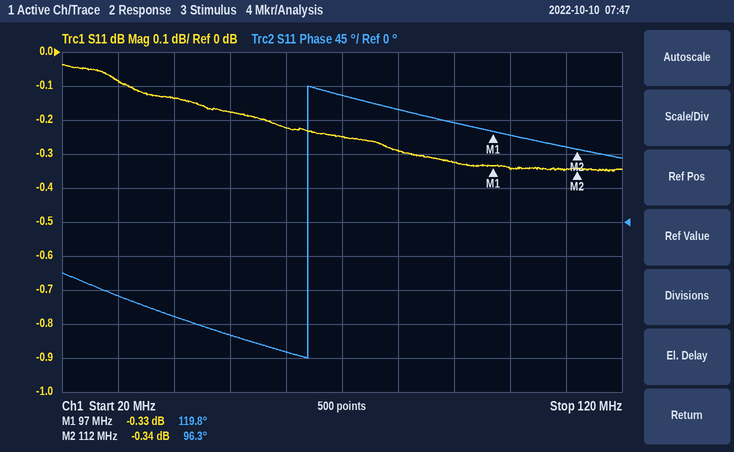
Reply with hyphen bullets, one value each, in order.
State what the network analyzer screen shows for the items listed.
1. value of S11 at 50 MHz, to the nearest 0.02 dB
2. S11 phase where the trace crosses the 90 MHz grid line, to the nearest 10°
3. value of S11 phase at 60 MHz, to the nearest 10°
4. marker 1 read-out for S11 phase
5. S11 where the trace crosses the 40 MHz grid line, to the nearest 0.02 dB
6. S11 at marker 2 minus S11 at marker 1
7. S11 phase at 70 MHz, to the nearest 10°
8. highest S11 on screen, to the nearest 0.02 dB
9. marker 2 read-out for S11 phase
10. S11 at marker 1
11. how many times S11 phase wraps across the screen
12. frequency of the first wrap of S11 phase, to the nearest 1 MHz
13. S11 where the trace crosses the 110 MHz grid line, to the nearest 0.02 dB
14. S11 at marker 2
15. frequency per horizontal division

- -0.18 dB
- 130°
- -170°
- 119.8°
- -0.14 dB
- -0.01 dB
- 170°
- -0.04 dB
- 96.3°
- -0.33 dB
- 1
- 64 MHz
- -0.34 dB
- -0.34 dB
- 10 MHz
